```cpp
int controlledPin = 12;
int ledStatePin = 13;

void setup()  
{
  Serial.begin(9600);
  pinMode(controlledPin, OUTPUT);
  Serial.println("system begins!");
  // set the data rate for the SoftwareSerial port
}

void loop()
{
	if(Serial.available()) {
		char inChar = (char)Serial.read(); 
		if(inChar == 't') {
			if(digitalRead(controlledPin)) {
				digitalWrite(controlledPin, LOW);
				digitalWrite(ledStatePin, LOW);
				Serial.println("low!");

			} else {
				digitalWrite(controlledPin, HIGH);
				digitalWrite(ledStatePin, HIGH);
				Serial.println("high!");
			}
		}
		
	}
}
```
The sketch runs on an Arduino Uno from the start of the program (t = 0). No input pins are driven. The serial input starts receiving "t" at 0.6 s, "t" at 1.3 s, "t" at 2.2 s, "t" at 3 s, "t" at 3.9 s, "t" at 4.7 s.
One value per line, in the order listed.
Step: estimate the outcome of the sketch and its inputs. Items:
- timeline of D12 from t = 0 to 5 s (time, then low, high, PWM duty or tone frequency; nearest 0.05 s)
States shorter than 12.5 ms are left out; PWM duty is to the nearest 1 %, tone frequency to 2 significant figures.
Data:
0 s low; 0.6 s high; 1.3 s low; 2.2 s high; 3 s low; 3.9 s high; 4.7 s low
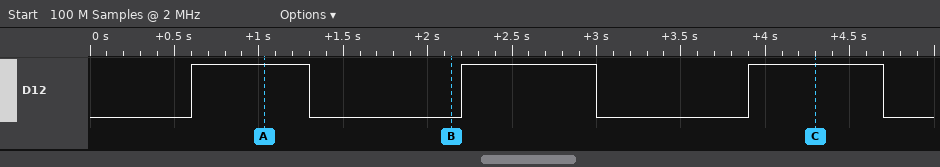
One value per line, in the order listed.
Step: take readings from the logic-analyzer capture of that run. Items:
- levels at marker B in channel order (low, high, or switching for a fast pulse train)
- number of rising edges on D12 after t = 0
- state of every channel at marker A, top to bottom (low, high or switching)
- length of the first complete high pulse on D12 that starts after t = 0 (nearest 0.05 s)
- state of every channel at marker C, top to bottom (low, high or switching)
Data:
D12 low
3
D12 high
0.70 s
D12 high
